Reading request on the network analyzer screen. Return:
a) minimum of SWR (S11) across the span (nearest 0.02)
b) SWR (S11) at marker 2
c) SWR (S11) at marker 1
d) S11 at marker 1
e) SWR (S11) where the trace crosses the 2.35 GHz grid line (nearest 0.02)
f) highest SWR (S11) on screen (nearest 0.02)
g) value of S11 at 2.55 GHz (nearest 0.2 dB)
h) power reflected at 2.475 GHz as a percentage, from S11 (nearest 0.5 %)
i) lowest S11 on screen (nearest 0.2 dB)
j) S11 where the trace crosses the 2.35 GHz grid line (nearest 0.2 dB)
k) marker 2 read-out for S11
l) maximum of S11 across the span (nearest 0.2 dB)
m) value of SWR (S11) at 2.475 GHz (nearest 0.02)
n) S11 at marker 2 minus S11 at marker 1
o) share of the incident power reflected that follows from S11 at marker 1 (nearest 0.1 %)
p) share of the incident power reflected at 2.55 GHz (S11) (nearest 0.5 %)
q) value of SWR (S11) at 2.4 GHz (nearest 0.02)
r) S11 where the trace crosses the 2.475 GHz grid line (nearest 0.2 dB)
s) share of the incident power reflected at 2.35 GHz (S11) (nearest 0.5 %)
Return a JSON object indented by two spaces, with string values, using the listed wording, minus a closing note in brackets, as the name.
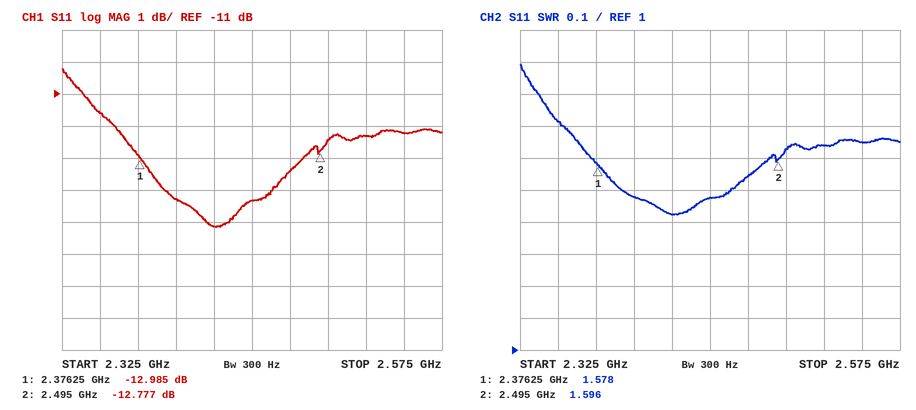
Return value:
{
  "minimum of SWR (S11) across the span": "1.42",
  "SWR (S11) at marker 2": "1.596",
  "SWR (S11) at marker 1": "1.578",
  "S11 at marker 1": "-12.985 dB",
  "SWR (S11) where the trace crosses the 2.35 GHz grid line": "1.72",
  "highest SWR (S11) on screen": "1.90",
  "value of S11 at 2.55 GHz": "-12.2 dB",
  "power reflected at 2.475 GHz as a percentage, from S11": "4.5 %",
  "lowest S11 on screen": "-15.2 dB",
  "S11 where the trace crosses the 2.35 GHz grid line": "-11.6 dB",
  "marker 2 read-out for S11": "-12.777 dB",
  "maximum of S11 across the span": "-10.2 dB",
  "value of SWR (S11) at 2.475 GHz": "1.54",
  "S11 at marker 2 minus S11 at marker 1": "0.208 dB",
  "share of the incident power reflected that follows from S11 at marker 1": "5.0 %",
  "share of the incident power reflected at 2.55 GHz (S11)": "6.0 %",
  "value of SWR (S11) at 2.4 GHz": "1.48",
  "S11 where the trace crosses the 2.475 GHz grid line": "-13.4 dB",
  "share of the incident power reflected at 2.35 GHz (S11)": "7.0 %"
}
